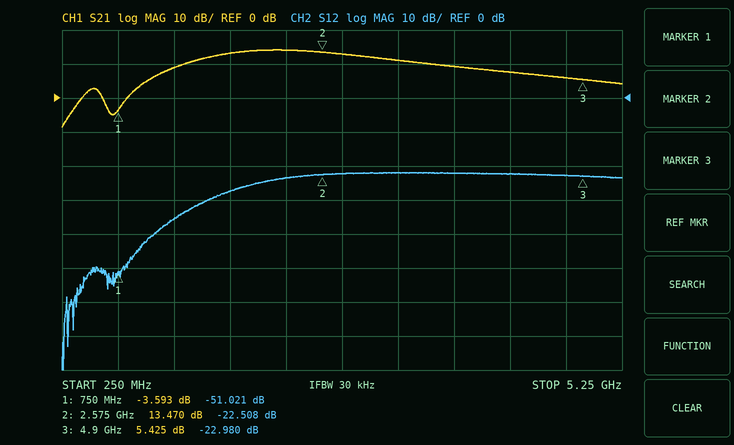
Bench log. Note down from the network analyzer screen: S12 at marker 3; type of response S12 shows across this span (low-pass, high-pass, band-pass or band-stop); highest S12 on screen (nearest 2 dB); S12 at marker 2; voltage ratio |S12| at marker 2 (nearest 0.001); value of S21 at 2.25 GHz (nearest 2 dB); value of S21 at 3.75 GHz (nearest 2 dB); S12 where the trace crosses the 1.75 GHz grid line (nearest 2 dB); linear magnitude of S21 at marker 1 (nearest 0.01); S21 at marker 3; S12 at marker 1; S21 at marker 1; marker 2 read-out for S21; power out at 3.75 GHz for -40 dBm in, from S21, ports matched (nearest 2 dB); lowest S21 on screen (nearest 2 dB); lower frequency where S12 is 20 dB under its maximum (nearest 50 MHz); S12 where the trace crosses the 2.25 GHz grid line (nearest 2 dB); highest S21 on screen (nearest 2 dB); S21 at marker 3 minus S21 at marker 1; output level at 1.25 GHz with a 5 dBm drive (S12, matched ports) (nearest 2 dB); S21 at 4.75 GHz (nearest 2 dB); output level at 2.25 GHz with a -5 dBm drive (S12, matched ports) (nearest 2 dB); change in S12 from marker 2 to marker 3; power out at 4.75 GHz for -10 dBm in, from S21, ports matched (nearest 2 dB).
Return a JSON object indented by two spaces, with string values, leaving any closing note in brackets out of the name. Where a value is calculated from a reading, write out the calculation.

{
  "S12 at marker 3": "-22.980 dB",
  "type of response S12 shows across this span": "high-pass",
  "highest S12 on screen": "-22 dB",
  "S12 at marker 2": "-22.508 dB",
  "voltage ratio |S12| at marker 2": "10^(-22.508/20) ≈ 0.075",
  "value of S21 at 2.25 GHz": "14 dB",
  "value of S21 at 3.75 GHz": "10 dB",
  "S12 where the trace crosses the 1.75 GHz grid line": "-28 dB",
  "linear magnitude of S21 at marker 1": "10^(-3.593/20) ≈ 0.66",
  "S21 at marker 3": "5.425 dB",
  "S12 at marker 1": "-51.021 dB",
  "S21 at marker 1": "-3.593 dB",
  "marker 2 read-out for S21": "13.470 dB",
  "power out at 3.75 GHz for -40 dBm in, from S21, ports matched": "-40 dBm + (10 dB) = -30 dBm",
  "lowest S21 on screen": "-8 dB",
  "lower frequency where S12 is 20 dB under its maximum": "1.00 GHz",
  "S12 where the trace crosses the 2.25 GHz grid line": "-24 dB",
  "highest S21 on screen": "14 dB",
  "S21 at marker 3 minus S21 at marker 1": "5.425 − (-3.593) = 9.018 dB",
  "output level at 1.25 GHz with a 5 dBm drive (S12, matched ports)": "5 dBm + (-36 dB) = -30 dBm",
  "S21 at 4.75 GHz": "6 dB",
  "output level at 2.25 GHz with a -5 dBm drive (S12, matched ports)": "-5 dBm + (-24 dB) = -28 dBm",
  "change in S12 from marker 2 to marker 3": "-22.98 − (-22.508) = -0.472 dB",
  "power out at 4.75 GHz for -10 dBm in, from S21, ports matched": "-10 dBm + (6 dB) = -4 dBm"
}
